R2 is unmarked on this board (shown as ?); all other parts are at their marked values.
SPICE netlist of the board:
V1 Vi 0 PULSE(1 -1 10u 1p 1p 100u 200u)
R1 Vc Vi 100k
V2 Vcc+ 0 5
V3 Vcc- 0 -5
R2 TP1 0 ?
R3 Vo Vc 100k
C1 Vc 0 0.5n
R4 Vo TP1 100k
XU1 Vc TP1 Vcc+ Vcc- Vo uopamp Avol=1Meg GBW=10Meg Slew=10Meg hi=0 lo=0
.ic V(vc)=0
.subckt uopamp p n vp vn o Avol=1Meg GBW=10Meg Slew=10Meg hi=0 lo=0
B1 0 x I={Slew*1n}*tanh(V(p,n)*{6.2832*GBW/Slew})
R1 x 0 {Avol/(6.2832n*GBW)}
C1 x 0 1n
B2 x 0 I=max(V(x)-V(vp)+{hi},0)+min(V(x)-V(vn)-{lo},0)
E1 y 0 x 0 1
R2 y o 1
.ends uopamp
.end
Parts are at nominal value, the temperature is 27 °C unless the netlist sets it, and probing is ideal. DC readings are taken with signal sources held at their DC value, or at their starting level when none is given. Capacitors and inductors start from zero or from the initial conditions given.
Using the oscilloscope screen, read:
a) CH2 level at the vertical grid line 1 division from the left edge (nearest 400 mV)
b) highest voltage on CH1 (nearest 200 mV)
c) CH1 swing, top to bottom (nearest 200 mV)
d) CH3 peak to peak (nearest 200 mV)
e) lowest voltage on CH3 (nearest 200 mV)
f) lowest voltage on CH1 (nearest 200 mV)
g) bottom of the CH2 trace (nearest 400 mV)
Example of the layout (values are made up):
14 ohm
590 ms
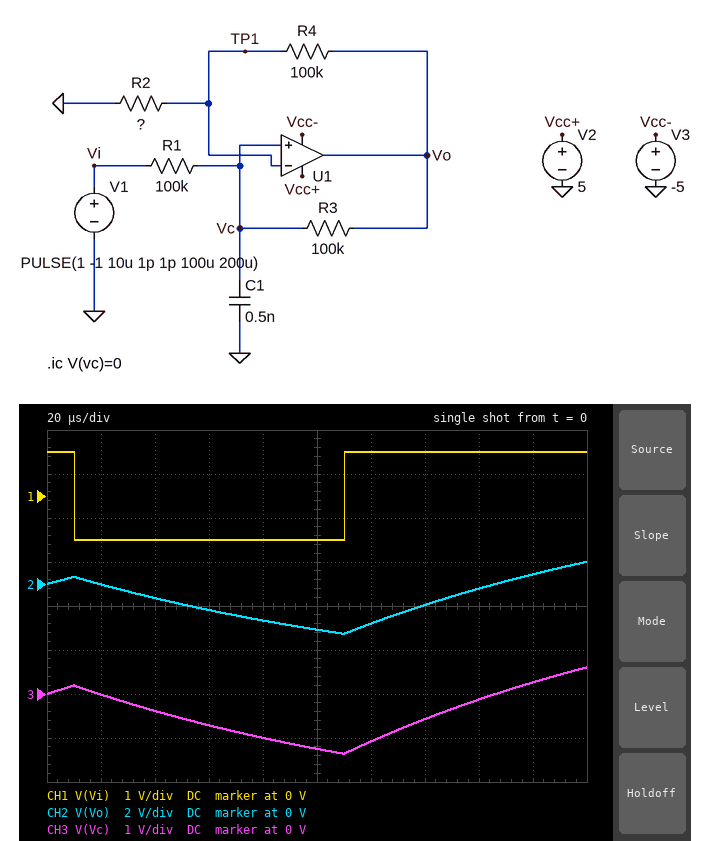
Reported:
0 V
1.0 V
2.0 V
2.0 V
-1.4 V
-1.0 V
-2.4 V
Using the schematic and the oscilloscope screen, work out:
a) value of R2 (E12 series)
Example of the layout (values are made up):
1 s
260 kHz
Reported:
150 kΩ
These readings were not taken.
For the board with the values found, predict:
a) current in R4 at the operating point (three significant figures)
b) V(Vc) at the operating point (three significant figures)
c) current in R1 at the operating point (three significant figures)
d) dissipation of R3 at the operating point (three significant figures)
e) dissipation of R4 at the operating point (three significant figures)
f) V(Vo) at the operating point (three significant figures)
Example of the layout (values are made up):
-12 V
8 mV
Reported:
20.0 µA
3.00 V
20.0 µA
40.0 µW
40.0 µW
5.00 V
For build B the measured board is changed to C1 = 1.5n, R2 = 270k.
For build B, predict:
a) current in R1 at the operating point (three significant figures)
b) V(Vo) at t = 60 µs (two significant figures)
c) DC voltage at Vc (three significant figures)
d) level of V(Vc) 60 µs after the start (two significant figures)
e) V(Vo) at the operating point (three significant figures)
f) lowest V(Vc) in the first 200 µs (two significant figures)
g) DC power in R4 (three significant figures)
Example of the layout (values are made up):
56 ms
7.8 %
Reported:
5.88 µA
-340 mV
1.59 V
-250 mV
2.18 V
-500 mV
3.46 µW
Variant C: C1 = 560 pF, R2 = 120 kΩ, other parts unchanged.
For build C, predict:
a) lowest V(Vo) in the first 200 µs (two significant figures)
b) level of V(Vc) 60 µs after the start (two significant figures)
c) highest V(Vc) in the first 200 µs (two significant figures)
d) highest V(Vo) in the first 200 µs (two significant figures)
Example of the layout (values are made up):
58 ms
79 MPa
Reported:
-2.6 V
-680 mV
330 mV
600 mV
